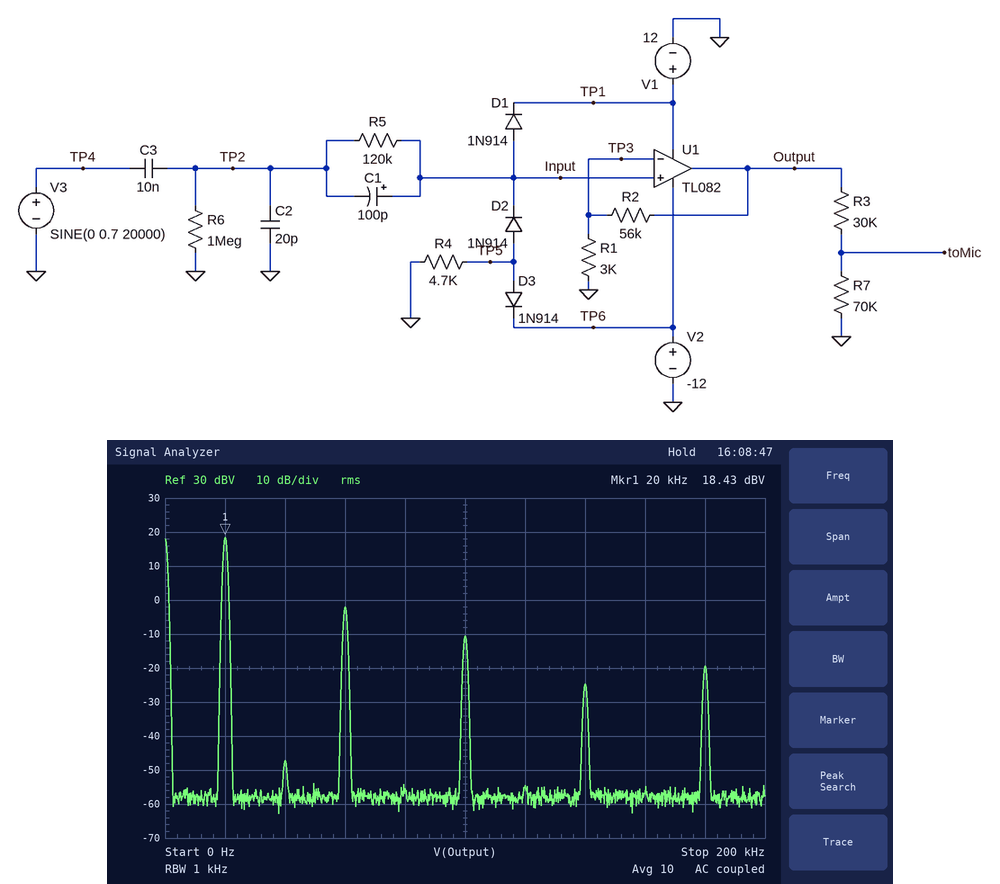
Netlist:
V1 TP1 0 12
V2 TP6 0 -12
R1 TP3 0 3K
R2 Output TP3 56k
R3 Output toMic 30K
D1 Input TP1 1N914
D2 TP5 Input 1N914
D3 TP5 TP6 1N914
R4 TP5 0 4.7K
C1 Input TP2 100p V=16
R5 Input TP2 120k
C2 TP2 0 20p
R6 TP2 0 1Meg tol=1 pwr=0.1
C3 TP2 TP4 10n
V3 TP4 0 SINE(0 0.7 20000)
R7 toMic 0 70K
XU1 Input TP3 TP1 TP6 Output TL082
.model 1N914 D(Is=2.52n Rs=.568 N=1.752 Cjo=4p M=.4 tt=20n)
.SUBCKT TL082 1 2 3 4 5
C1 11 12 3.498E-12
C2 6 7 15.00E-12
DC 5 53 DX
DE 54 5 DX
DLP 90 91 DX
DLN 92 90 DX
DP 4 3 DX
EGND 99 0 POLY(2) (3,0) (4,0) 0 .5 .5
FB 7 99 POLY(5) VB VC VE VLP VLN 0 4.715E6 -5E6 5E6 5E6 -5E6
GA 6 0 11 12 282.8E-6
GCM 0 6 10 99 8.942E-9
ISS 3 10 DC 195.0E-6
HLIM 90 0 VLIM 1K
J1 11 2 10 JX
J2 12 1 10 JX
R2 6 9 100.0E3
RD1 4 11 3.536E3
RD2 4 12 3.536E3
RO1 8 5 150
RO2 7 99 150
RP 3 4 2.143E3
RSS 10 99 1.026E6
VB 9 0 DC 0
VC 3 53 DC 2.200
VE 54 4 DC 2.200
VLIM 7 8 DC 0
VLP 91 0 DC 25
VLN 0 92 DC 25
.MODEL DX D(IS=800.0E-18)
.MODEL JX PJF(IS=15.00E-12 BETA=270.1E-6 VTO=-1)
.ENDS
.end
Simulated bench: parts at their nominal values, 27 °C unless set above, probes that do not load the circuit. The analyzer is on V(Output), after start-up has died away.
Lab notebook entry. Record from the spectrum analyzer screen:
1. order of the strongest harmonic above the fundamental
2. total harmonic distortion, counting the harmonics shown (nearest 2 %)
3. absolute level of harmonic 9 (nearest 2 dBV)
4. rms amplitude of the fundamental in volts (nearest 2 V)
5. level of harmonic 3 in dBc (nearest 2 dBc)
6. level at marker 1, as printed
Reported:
3
10 %
-20 dBV
8 V
-20 dBc
18.43 dBV
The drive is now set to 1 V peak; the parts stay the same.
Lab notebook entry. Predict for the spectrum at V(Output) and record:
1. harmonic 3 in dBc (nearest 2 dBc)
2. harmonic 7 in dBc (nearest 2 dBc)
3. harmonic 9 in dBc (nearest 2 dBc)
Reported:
-14 dBc
-32 dBc
-32 dBc
